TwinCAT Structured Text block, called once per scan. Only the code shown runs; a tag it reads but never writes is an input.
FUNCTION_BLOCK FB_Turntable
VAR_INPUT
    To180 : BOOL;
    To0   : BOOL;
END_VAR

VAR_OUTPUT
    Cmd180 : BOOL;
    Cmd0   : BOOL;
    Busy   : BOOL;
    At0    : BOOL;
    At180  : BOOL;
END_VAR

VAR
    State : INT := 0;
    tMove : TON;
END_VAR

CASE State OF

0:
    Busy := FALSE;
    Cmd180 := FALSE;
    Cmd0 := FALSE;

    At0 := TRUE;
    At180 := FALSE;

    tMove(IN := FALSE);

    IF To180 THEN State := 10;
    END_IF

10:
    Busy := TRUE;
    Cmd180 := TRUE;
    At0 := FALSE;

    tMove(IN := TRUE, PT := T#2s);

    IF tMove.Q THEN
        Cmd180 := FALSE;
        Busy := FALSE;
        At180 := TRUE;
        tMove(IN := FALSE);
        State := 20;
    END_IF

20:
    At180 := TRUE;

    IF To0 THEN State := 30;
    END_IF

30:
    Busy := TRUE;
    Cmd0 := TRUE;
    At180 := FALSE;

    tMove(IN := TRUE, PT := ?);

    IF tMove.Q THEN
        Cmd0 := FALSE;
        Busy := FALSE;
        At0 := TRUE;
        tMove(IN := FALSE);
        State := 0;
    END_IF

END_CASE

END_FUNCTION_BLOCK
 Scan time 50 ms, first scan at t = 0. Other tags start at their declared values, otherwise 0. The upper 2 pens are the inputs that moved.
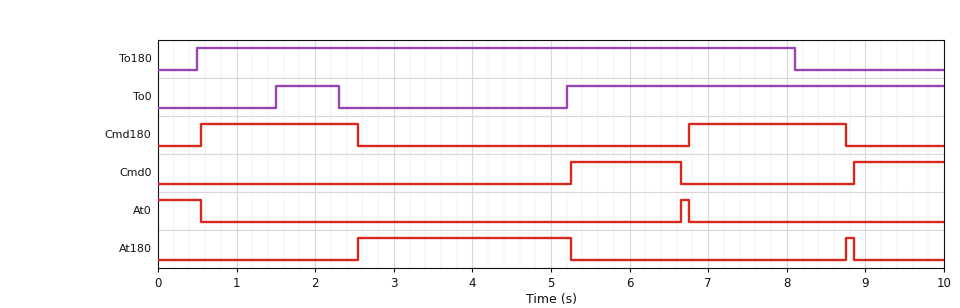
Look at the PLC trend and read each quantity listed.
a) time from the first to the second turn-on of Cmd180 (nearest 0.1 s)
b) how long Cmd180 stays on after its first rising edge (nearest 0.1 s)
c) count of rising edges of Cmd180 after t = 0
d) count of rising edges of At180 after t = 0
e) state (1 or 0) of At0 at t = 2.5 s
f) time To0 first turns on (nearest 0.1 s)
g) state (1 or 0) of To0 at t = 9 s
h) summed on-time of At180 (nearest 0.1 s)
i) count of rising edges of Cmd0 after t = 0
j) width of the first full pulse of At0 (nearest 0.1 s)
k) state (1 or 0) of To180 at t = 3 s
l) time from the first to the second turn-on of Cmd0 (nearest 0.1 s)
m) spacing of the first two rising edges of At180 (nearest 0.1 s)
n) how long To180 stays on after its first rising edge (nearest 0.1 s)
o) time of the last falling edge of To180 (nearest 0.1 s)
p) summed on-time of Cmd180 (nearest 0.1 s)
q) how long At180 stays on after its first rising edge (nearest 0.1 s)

6.2 s
2.0 s
2
2
0
1.5 s
1
2.8 s
2
0.1 s
1
3.6 s
6.2 s
7.6 s
8.1 s
4.0 s
2.7 s
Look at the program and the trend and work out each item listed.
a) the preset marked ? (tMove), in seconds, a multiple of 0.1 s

1.4 s
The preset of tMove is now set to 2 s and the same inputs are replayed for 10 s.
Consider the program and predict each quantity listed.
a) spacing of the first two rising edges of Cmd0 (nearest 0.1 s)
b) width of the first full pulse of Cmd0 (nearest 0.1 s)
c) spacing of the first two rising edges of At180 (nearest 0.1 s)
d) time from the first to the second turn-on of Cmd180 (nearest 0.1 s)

4.2 s
2.0 s
6.8 s
6.8 s
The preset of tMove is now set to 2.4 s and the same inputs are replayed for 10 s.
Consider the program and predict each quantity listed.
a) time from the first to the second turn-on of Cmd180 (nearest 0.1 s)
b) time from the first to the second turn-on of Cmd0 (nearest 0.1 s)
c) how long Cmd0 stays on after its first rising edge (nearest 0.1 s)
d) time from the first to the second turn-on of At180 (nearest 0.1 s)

7.2 s
4.6 s
2.4 s
7.2 s
